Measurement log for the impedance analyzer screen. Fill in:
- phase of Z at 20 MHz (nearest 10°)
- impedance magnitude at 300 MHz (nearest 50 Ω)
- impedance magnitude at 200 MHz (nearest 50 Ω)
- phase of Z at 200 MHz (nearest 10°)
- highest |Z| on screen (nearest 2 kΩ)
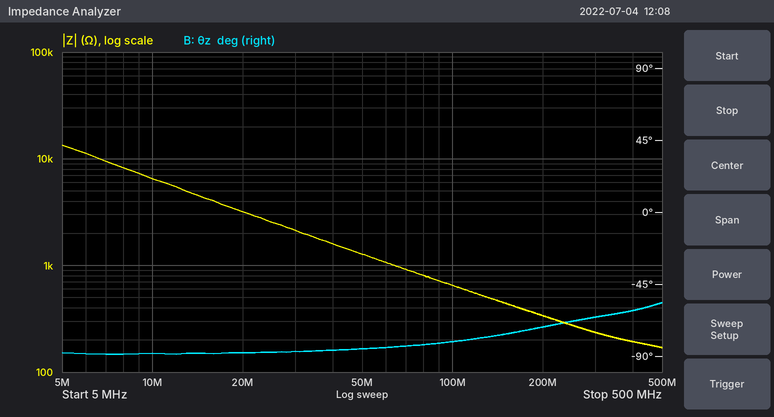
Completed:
-90°
250 Ω
350 Ω
-70°
14 kΩ
